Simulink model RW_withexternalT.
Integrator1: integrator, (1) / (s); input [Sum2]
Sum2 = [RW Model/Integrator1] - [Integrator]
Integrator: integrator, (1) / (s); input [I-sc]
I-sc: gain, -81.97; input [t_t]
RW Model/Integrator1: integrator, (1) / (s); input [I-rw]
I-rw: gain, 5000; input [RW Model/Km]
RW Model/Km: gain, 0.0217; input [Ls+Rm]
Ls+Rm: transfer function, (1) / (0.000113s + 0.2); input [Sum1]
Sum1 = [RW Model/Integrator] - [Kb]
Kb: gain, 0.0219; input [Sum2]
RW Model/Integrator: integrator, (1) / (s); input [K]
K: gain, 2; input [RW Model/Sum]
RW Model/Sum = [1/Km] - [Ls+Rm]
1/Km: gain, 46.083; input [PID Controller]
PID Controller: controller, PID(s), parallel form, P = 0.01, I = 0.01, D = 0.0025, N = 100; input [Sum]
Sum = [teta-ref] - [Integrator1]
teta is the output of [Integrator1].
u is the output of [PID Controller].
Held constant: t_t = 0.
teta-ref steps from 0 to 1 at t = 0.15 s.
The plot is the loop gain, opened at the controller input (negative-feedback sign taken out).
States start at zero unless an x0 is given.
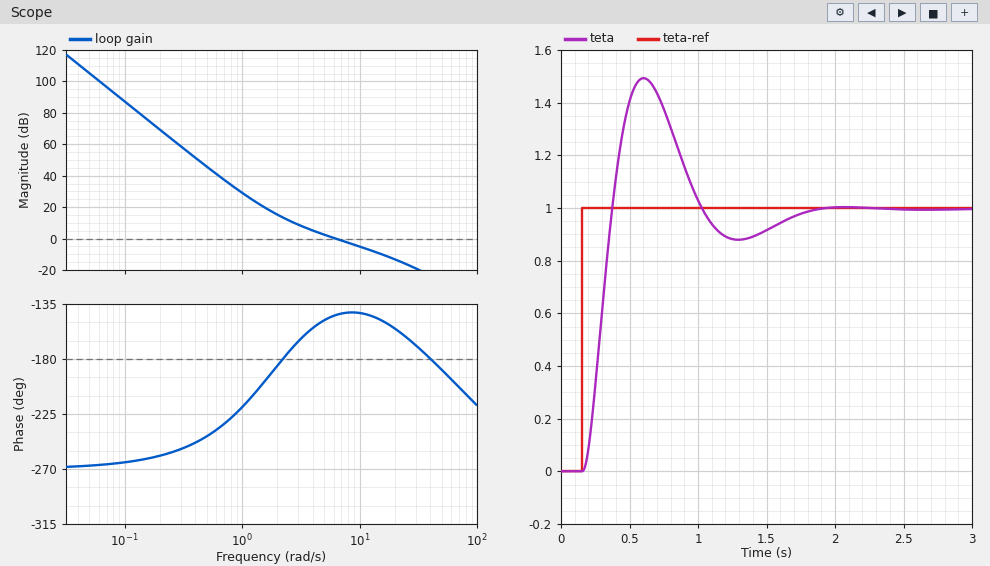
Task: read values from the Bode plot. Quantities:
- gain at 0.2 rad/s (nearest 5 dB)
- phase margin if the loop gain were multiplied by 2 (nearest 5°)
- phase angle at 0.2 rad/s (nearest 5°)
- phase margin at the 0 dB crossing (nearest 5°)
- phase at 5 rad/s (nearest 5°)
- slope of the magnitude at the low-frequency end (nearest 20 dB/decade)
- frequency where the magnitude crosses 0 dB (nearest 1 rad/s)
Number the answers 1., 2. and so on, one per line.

1. 70 dB
2. 35°
3. -260°
4. 35°
5. -150°
6. -60 dB/decade
7. 6 rad/s
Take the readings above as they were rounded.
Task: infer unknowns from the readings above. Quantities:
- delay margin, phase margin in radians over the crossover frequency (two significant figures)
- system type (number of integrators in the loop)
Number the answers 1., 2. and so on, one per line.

1. 0.10 s
2. 3
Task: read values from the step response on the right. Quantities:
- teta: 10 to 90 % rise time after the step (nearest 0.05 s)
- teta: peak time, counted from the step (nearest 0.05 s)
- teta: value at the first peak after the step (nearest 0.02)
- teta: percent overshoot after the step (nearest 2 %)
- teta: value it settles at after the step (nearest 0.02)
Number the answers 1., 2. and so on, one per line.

1. 0.15 s
2. 0.45 s
3. 1.50
4. 50 %
5. 1.00
